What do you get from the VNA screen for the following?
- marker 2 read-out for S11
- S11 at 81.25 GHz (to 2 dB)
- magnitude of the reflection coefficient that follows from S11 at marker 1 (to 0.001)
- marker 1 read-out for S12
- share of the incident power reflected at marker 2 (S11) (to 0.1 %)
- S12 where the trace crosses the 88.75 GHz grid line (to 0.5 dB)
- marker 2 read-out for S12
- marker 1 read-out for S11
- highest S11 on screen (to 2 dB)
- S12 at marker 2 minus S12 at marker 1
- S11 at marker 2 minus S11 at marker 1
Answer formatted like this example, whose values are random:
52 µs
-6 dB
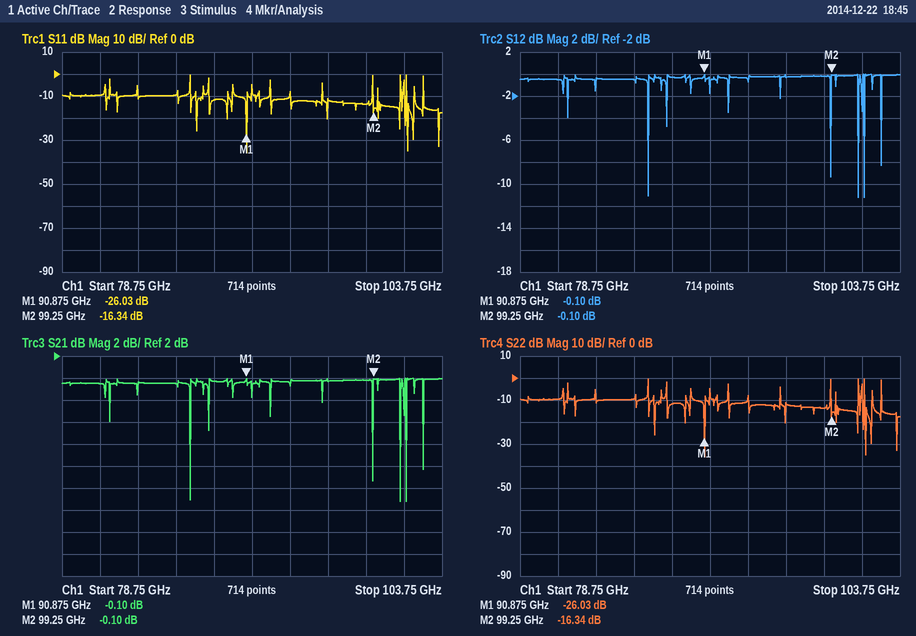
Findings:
-16.34 dB
-10 dB
0.050
-0.10 dB
2.3 %
-0.5 dB
-0.10 dB
-26.03 dB
0 dB
0.00 dB
9.69 dB
